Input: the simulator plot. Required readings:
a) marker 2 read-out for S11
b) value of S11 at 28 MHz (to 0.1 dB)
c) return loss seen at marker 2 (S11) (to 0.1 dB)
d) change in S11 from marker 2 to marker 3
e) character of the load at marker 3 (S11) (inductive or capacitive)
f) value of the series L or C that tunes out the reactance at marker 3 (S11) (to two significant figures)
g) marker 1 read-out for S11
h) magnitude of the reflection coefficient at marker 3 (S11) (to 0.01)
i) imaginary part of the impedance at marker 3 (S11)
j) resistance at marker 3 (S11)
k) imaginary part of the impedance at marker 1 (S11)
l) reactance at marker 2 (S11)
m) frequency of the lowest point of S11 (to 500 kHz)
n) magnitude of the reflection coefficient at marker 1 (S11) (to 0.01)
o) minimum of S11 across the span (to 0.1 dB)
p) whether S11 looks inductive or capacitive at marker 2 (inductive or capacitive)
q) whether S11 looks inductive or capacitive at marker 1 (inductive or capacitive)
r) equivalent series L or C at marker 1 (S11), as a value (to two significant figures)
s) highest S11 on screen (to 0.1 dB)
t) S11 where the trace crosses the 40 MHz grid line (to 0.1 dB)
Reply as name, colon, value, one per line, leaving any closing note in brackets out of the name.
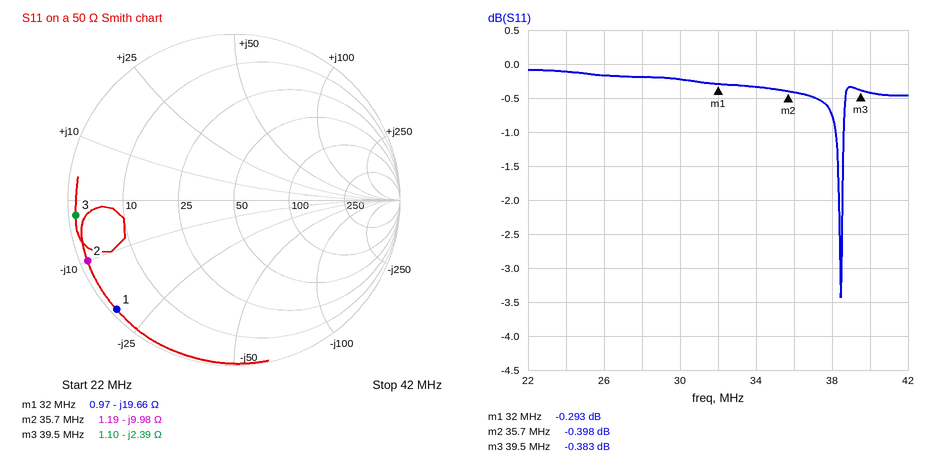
marker 2 read-out for S11: -0.398 dB
value of S11 at 28 MHz: -0.2 dB
return loss seen at marker 2 (S11): 0.4 dB
change in S11 from marker 2 to marker 3: 0.015 dB
character of the load at marker 3 (S11): capacitive
value of the series L or C that tunes out the reactance at marker 3 (S11): 9.6 nH
marker 1 read-out for S11: -0.293 dB
magnitude of the reflection coefficient at marker 3 (S11): 0.96
imaginary part of the impedance at marker 3: -2.39 Ω
resistance at marker 3: 1.10 Ω
imaginary part of the impedance at marker 1: -19.66 Ω
reactance at marker 2: -9.98 Ω
frequency of the lowest point of S11: 38.5 MHz
magnitude of the reflection coefficient at marker 1 (S11): 0.97
minimum of S11 across the span: -3.4 dB
whether S11 looks inductive or capacitive at marker 2: capacitive
whether S11 looks inductive or capacitive at marker 1: capacitive
equivalent series L or C at marker 1 (S11), as a value: 250 pF
highest S11 on screen: -0.1 dB
S11 where the trace crosses the 40 MHz grid line: -0.4 dB
